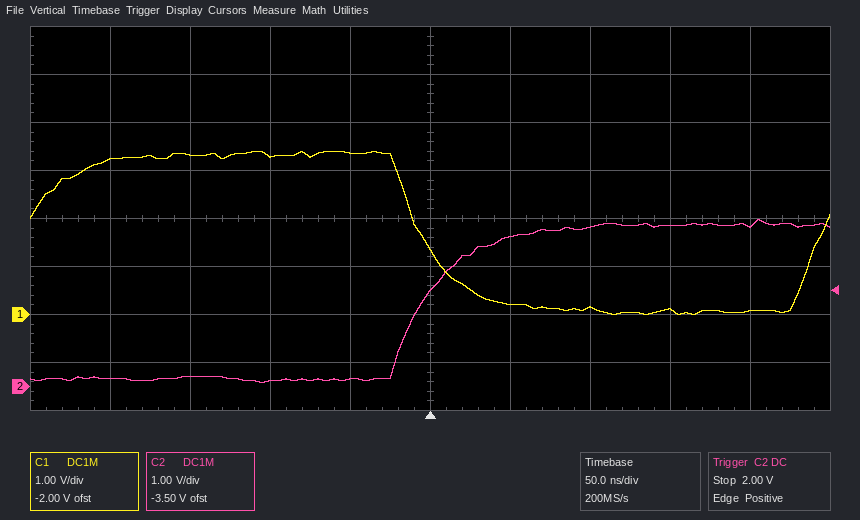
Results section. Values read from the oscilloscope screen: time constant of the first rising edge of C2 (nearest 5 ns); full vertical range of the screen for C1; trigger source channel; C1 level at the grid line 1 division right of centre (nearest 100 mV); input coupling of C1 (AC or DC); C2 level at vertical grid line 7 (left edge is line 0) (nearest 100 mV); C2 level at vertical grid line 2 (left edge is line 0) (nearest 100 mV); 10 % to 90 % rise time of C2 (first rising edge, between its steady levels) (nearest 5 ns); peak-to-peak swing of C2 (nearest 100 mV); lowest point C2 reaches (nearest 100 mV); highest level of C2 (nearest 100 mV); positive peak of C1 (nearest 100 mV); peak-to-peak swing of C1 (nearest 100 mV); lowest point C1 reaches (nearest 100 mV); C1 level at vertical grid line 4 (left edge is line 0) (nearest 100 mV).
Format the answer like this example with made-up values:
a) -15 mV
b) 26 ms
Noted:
a) 30 ns
b) 8 V
c) C2
d) 200 mV
e) DC
f) 3.3 V
g) 200 mV
h) 65 ns
i) 3.4 V
j) 100 mV
k) 3.5 V
l) 3.4 V
m) 3.4 V
n) 0.0 V
o) 3.4 V
